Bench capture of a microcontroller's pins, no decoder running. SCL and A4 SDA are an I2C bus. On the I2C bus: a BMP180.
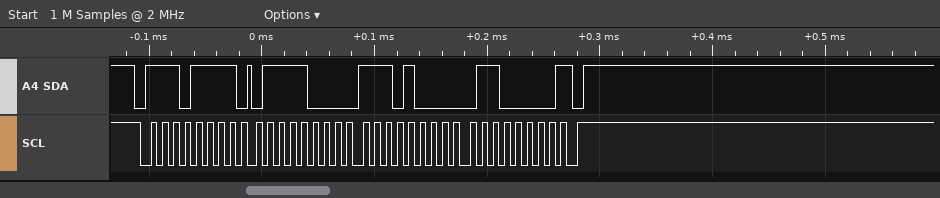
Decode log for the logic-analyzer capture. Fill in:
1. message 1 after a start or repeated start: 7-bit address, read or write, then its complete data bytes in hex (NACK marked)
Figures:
0x77 read: 78 E8 60 NACK
